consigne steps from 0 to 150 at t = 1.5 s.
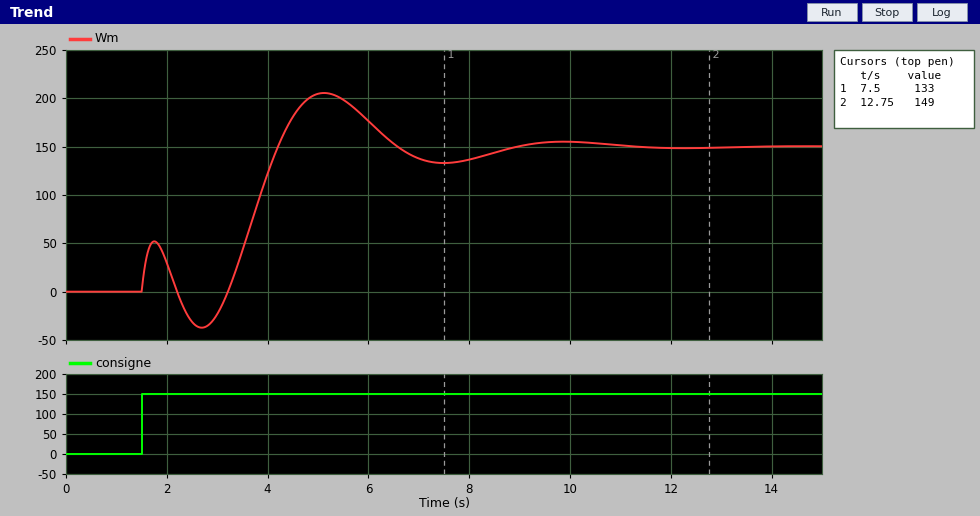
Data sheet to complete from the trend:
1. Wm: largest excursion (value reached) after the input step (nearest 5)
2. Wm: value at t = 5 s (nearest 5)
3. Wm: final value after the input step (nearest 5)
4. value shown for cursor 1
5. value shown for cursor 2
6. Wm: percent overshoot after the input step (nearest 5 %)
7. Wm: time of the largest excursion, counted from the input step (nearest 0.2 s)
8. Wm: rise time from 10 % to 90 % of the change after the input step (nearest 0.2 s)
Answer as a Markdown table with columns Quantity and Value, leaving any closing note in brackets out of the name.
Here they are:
| Quantity | Value |
|---|---|
| Wm: largest excursion (value reached) after the input step | 205 |
| Wm: value at t = 5 s | 205 |
| Wm: final value after the input step | 150 |
| value shown for cursor 1 | 133 |
| value shown for cursor 2 | 149 |
| Wm: percent overshoot after the input step | 35 % |
| Wm: time of the largest excursion, counted from the input step | 3.6 s |
| Wm: rise time from 10 % to 90 % of the change after the input step | 2.6 s |
